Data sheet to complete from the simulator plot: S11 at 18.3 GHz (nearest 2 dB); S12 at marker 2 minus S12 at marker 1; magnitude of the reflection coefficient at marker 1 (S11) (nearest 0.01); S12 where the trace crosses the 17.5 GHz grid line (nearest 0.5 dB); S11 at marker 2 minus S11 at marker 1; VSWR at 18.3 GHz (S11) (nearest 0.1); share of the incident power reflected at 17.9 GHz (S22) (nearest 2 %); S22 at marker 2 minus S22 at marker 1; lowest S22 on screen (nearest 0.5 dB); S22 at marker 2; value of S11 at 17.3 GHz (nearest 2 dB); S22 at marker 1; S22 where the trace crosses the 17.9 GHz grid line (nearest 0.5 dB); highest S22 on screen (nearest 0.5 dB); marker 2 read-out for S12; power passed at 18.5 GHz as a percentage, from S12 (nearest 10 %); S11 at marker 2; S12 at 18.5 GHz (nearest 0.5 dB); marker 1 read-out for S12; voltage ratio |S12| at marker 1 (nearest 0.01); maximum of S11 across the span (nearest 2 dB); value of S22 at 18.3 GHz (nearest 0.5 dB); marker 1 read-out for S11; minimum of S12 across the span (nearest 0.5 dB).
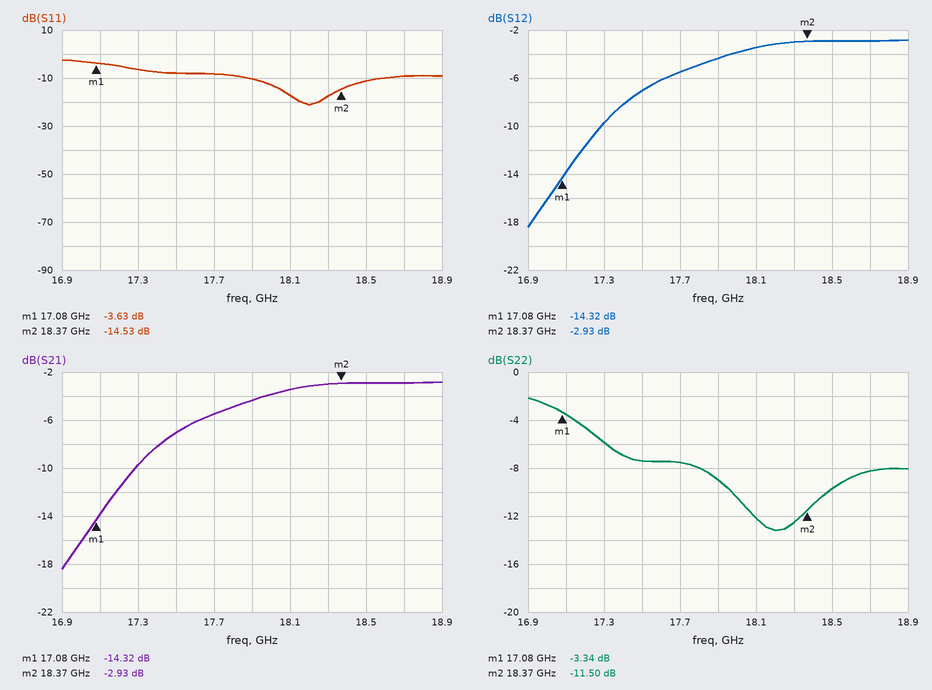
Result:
-18 dB
11.39 dB
0.66
-7.0 dB
-10.90 dB
1.3
12 %
-8.16 dB
-13.0 dB
-11.50 dB
-6 dB
-3.34 dB
-9.0 dB
-2.0 dB
-2.93 dB
50 %
-14.53 dB
-3.0 dB
-14.32 dB
0.19
-2 dB
-12.5 dB
-3.63 dB
-18.5 dB
